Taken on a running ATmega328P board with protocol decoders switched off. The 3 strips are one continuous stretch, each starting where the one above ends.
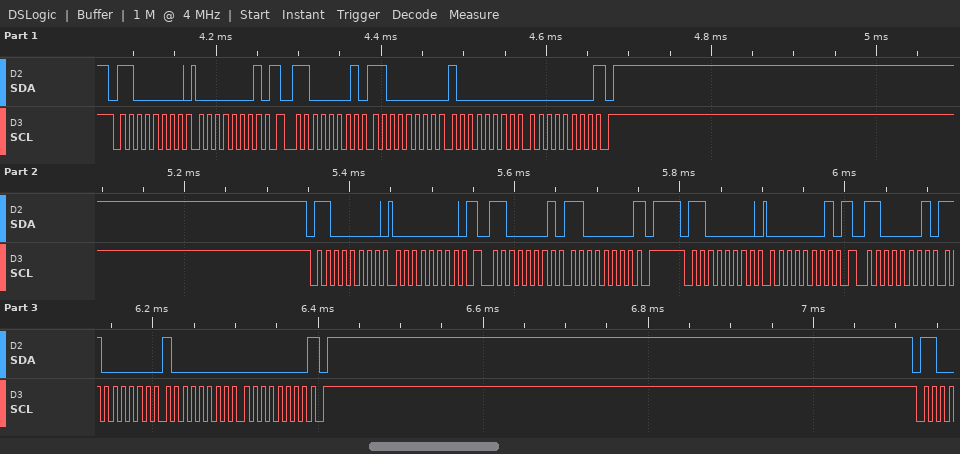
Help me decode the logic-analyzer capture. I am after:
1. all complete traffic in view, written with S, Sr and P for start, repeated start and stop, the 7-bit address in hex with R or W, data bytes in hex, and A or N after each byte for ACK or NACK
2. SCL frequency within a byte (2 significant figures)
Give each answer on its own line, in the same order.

S 60W A 01 A Sr 60R A C0 A 80 A 00 N P S 60W A 00 A Sr 60R A C0 N P S 60W A 01 A Sr 60R A C0 A 80 A 00 N P
100 kHz
